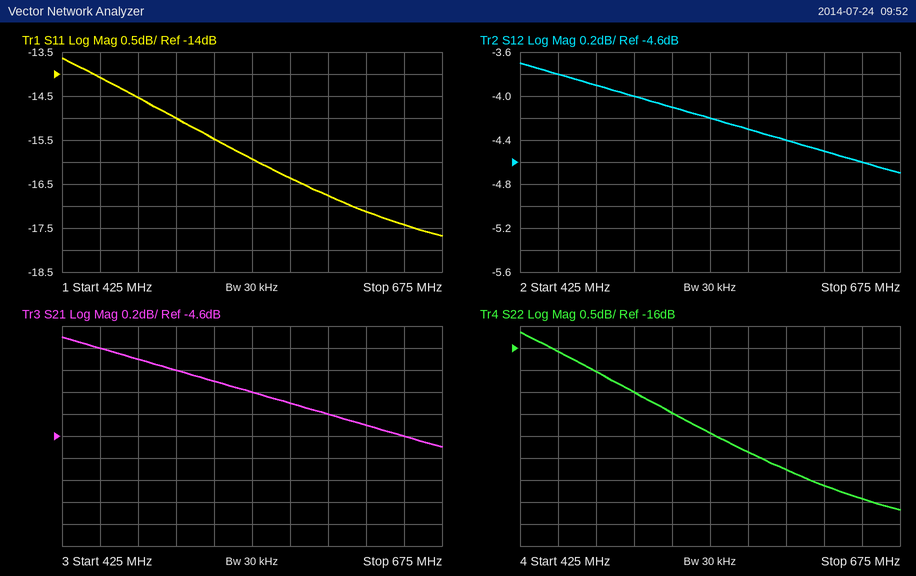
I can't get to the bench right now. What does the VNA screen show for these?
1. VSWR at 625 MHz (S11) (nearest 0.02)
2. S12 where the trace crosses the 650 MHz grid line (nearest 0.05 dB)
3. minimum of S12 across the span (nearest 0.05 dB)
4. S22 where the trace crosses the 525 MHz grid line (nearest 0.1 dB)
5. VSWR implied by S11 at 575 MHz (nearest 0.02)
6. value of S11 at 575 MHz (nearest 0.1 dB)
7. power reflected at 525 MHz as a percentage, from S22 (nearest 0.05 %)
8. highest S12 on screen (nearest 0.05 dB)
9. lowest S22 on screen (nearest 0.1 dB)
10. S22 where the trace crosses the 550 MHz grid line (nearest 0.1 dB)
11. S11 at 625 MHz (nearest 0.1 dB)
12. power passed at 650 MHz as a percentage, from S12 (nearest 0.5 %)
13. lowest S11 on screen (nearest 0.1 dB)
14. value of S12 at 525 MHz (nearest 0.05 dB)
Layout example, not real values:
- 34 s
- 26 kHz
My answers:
- 1.32
- -4.60 dB
- -4.70 dB
- -17.5 dB
- 1.36
- -16.4 dB
- 1.80 %
- -3.70 dB
- -19.7 dB
- -17.9 dB
- -17.1 dB
- 34.5 %
- -17.7 dB
- -4.10 dB
